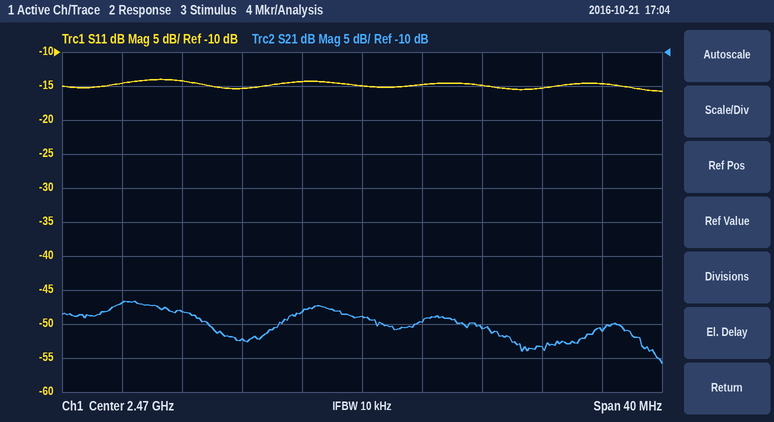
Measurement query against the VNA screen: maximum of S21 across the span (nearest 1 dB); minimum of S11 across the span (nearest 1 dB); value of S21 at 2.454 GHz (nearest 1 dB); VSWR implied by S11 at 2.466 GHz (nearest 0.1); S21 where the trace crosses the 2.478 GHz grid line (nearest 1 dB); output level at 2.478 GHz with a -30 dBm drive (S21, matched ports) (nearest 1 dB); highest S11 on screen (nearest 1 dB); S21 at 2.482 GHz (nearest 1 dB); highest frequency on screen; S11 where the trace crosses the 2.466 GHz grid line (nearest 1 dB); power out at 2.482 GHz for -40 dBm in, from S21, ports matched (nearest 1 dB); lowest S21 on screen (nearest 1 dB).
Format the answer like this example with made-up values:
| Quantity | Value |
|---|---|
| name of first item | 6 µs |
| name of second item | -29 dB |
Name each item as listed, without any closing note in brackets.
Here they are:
| Quantity | Value |
|---|---|
| maximum of S21 across the span | -47 dB |
| minimum of S11 across the span | -16 dB |
| value of S21 at 2.454 GHz | -47 dB |
| VSWR implied by S11 at 2.466 GHz | 1.5 |
| S21 where the trace crosses the 2.478 GHz grid line | -51 dB |
| output level at 2.478 GHz with a -30 dBm drive (S21, matched ports) | -81 dBm |
| highest S11 on screen | -14 dB |
| S21 at 2.482 GHz | -53 dB |
| highest frequency on screen | 2.49 GHz |
| S11 where the trace crosses the 2.466 GHz grid line | -14 dB |
| power out at 2.482 GHz for -40 dBm in, from S21, ports matched | -93 dBm |
| lowest S21 on screen | -56 dB |
